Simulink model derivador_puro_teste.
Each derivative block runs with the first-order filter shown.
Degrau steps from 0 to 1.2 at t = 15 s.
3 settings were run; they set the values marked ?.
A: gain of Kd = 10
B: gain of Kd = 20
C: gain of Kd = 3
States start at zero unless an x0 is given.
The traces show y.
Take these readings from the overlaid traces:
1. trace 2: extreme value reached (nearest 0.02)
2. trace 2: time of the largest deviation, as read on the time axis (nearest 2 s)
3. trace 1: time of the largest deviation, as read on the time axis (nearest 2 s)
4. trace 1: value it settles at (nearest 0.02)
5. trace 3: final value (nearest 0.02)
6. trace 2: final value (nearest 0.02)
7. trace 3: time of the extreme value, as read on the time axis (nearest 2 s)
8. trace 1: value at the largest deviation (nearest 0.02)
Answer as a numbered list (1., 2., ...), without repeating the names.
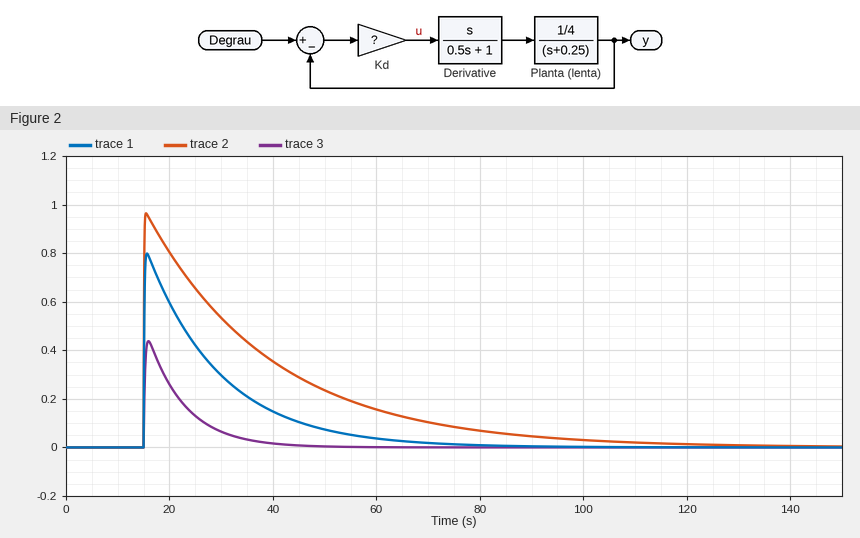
1. 0.96
2. 16 s
3. 16 s
4. 0.00
5. 0.00
6. 0.00
7. 16 s
8. 0.80
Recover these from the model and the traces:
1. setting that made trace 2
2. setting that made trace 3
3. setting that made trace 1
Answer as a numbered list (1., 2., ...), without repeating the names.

1. B
2. C
3. A
